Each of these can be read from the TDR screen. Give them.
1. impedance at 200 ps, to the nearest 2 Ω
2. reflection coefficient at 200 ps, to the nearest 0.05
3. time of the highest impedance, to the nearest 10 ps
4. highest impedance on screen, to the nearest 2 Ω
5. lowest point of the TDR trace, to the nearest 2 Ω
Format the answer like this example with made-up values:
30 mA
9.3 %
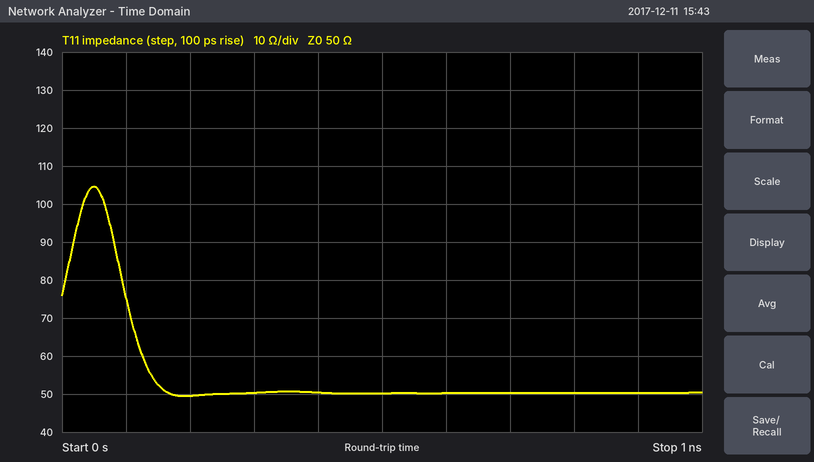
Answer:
50 Ω
0.00
50 ps
104 Ω
50 Ω
